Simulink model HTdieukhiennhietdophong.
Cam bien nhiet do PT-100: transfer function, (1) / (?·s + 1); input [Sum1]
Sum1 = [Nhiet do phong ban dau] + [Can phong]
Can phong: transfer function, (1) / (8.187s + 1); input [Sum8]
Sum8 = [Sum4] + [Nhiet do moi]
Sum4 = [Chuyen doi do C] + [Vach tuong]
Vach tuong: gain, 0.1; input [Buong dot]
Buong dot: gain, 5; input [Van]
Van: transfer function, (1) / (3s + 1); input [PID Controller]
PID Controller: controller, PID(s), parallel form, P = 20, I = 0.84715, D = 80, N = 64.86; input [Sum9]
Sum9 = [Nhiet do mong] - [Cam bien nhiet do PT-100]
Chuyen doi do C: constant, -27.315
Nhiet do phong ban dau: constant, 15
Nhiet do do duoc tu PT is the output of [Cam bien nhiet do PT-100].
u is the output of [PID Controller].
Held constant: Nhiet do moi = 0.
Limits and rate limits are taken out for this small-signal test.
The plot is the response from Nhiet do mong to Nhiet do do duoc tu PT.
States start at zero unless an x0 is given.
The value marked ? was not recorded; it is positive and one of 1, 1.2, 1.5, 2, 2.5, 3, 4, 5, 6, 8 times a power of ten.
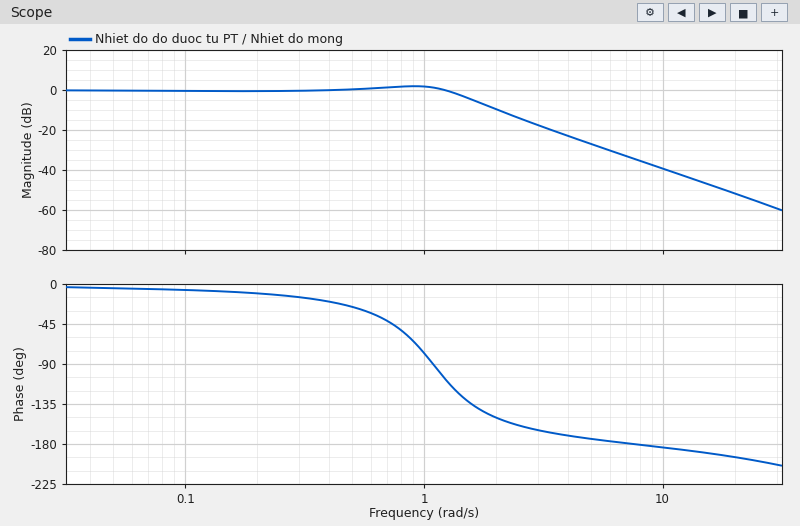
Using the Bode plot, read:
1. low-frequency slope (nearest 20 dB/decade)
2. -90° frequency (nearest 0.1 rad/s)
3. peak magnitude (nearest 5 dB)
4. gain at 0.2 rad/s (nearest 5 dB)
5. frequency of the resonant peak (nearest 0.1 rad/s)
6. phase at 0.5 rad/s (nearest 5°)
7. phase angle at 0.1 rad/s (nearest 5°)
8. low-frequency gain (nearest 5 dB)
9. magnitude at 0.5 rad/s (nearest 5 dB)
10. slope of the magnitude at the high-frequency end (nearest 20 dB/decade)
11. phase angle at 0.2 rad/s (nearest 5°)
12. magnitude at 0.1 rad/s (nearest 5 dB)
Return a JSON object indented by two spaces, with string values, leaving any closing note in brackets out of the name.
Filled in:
{
  "low-frequency slope": "0 dB/decade",
  "-90° frequency": "1.1 rad/s",
  "peak magnitude": "0 dB",
  "gain at 0.2 rad/s": "0 dB",
  "frequency of the resonant peak": "0.9 rad/s",
  "phase at 0.5 rad/s": "-25°",
  "phase angle at 0.1 rad/s": "-5°",
  "low-frequency gain": "0 dB",
  "magnitude at 0.5 rad/s": "0 dB",
  "slope of the magnitude at the high-frequency end": "-40 dB/decade",
  "phase angle at 0.2 rad/s": "-10°",
  "magnitude at 0.1 rad/s": "0 dB"
}
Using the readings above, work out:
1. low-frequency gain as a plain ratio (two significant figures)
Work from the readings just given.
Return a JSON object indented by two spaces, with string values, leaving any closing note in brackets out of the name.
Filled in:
{
  "low-frequency gain as a plain ratio": "1.0"
}
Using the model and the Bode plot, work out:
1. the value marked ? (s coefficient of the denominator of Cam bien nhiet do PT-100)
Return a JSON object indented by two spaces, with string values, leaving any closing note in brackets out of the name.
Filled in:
{
  "the value marked ?": "1.5"
}
